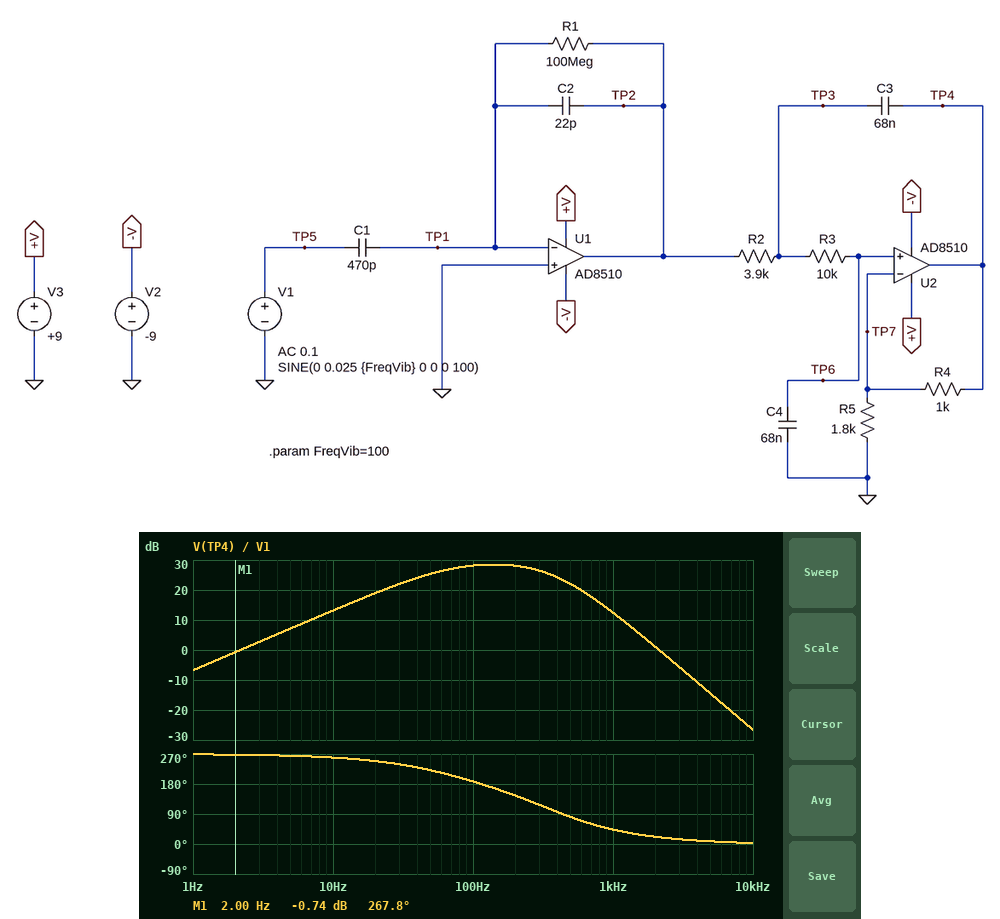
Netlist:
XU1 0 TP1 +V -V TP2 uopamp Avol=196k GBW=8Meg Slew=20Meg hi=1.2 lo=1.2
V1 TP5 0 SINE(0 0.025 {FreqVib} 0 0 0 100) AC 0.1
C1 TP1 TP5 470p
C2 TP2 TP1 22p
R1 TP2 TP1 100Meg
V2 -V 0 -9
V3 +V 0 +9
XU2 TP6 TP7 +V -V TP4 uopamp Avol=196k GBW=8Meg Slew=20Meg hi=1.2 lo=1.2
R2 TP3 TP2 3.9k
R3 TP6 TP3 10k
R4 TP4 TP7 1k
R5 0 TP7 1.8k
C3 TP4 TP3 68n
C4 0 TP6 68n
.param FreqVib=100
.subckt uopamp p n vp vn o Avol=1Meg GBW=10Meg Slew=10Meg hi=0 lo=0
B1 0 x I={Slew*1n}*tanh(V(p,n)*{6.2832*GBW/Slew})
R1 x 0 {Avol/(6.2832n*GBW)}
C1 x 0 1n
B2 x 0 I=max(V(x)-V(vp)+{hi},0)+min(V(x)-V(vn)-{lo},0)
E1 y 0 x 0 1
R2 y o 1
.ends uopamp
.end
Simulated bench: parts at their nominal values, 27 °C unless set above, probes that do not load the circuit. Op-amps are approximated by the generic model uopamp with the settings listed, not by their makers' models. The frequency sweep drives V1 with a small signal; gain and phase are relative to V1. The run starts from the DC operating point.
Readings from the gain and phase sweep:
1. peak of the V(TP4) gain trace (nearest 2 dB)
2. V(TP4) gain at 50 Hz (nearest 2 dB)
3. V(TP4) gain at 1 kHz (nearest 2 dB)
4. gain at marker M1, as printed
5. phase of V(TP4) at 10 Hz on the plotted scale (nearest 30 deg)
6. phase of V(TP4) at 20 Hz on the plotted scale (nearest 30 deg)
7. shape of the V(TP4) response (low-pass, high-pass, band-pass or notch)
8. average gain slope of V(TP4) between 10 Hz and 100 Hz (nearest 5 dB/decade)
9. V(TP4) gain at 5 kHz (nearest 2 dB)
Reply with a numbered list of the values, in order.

1. 28 dB
2. 26 dB
3. 12 dB
4. -0.74 dB
5. 270 deg
6. 240 deg
7. band-pass
8. 15 dB/decade
9. -14 dB
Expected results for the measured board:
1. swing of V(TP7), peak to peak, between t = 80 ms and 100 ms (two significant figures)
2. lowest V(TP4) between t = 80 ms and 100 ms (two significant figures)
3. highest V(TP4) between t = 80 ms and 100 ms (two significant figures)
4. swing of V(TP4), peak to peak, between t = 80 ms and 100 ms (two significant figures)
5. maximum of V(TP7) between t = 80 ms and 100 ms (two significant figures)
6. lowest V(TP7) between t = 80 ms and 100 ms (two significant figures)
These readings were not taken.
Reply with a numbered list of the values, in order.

1. 820 mV
2. -640 mV
3. 640 mV
4. 1.3 V
5. 410 mV
6. -410 mV
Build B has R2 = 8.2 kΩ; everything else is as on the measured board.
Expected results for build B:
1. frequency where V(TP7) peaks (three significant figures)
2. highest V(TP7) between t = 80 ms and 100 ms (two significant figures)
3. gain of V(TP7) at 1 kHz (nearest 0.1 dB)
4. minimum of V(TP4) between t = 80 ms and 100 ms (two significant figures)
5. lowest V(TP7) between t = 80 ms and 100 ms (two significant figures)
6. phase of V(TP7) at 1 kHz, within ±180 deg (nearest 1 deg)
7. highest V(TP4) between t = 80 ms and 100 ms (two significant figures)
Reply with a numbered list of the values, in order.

1. 139 Hz
2. 420 mV
3. 3.0 dB
4. -650 mV
5. -420 mV
6. 27 deg
7. 650 mV
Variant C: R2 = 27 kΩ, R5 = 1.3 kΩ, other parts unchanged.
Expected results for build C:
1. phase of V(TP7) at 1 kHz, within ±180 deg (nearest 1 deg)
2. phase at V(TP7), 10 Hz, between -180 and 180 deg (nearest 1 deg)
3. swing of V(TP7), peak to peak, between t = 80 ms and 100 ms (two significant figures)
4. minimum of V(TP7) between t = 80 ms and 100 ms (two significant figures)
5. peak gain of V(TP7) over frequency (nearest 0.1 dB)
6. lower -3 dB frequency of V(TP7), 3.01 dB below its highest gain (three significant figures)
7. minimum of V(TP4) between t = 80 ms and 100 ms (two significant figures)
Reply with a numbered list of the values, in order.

1. 12 deg
2. -102 deg
3. 1.0 V
4. -500 mV
5. 26.4 dB
6. 59.5 Hz
7. -890 mV
